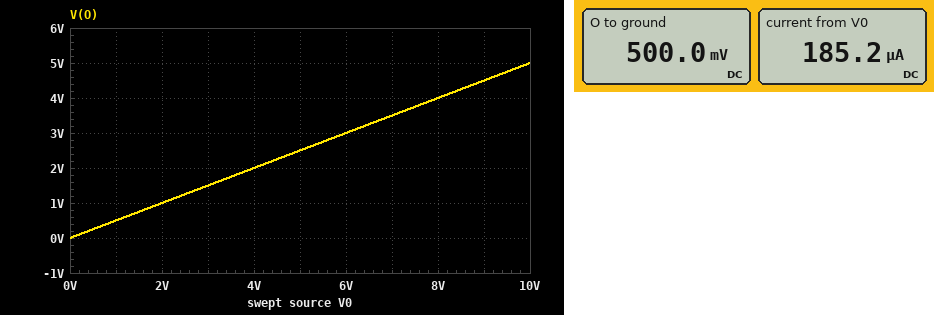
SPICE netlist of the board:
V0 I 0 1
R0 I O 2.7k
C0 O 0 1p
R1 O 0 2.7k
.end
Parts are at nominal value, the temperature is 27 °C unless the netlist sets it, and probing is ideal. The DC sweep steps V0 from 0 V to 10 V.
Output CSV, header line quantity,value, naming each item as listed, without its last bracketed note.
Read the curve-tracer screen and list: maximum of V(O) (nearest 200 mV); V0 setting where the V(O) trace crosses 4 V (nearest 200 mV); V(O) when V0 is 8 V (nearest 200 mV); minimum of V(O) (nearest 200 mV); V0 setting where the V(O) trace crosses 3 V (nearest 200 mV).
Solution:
quantity,value
maximum of V(O),5.0 V
V0 setting where the V(O) trace crosses 4 V,8.0 V
V(O) when V0 is 8 V,4.0 V
minimum of V(O),0 V
V0 setting where the V(O) trace crosses 3 V,6.0 V
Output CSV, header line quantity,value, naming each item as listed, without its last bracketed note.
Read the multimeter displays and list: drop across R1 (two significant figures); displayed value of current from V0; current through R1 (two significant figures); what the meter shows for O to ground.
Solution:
quantity,value
drop across R1,500 mV
displayed value of current from V0,185.2 µA
current through R1,190 µA
what the meter shows for O to ground,500.0 mV
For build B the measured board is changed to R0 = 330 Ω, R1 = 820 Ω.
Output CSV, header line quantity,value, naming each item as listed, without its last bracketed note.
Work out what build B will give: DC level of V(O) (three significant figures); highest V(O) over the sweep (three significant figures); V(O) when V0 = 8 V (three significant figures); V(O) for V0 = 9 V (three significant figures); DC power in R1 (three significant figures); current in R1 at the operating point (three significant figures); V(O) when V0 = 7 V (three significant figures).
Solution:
quantity,value
DC level of V(O),713 mV
highest V(O) over the sweep,7.13 V
V(O) when V0 = 8 V,5.70 V
V(O) for V0 = 9 V,6.42 V
DC power in R1,620 µW
current in R1 at the operating point,870 µA
V(O) when V0 = 7 V,4.99 V
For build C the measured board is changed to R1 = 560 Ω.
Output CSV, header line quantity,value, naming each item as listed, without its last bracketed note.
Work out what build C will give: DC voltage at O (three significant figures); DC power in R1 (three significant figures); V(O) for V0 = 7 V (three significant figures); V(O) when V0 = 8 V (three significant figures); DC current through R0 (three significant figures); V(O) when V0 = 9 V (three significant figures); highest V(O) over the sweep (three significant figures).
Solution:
quantity,value
DC voltage at O,172 mV
DC power in R1,52.7 µW
V(O) for V0 = 7 V,1.20 V
V(O) when V0 = 8 V,1.37 V
DC current through R0,307 µA
V(O) when V0 = 9 V,1.55 V
highest V(O) over the sweep,1.72 V
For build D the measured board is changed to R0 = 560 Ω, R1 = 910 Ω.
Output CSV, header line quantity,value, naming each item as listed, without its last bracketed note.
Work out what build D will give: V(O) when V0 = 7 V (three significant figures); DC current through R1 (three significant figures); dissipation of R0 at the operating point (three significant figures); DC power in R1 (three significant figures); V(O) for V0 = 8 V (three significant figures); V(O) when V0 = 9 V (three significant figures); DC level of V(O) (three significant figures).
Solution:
quantity,value
V(O) when V0 = 7 V,4.33 V
DC current through R1,680 µA
dissipation of R0 at the operating point,259 µW
DC power in R1,421 µW
V(O) for V0 = 8 V,4.95 V
V(O) when V0 = 9 V,5.57 V
DC level of V(O),619 mV
